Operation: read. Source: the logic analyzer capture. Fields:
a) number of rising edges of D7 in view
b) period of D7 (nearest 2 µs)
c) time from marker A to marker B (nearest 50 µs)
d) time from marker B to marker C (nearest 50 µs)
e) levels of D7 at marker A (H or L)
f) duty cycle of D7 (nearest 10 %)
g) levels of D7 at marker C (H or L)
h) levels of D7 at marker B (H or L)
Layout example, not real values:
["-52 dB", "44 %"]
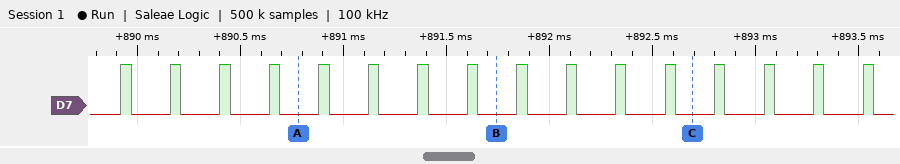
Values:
["16", "240 µs", "950 µs", "950 µs", "D7=L", "20 %", "D7=L", "D7=L"]
